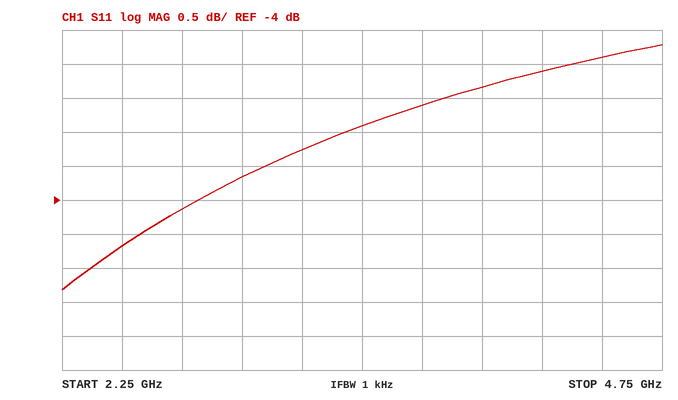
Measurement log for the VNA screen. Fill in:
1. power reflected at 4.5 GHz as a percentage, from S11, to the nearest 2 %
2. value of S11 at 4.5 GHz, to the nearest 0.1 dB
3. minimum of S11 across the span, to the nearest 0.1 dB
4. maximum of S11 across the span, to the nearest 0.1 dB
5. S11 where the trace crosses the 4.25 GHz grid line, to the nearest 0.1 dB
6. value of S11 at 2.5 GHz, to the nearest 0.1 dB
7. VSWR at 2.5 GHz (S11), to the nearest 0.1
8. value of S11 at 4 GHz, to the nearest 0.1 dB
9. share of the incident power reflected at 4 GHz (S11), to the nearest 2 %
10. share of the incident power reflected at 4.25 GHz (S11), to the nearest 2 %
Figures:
64 %
-1.9 dB
-5.3 dB
-1.7 dB
-2.1 dB
-4.7 dB
3.8
-2.3 dB
58 %
62 %
